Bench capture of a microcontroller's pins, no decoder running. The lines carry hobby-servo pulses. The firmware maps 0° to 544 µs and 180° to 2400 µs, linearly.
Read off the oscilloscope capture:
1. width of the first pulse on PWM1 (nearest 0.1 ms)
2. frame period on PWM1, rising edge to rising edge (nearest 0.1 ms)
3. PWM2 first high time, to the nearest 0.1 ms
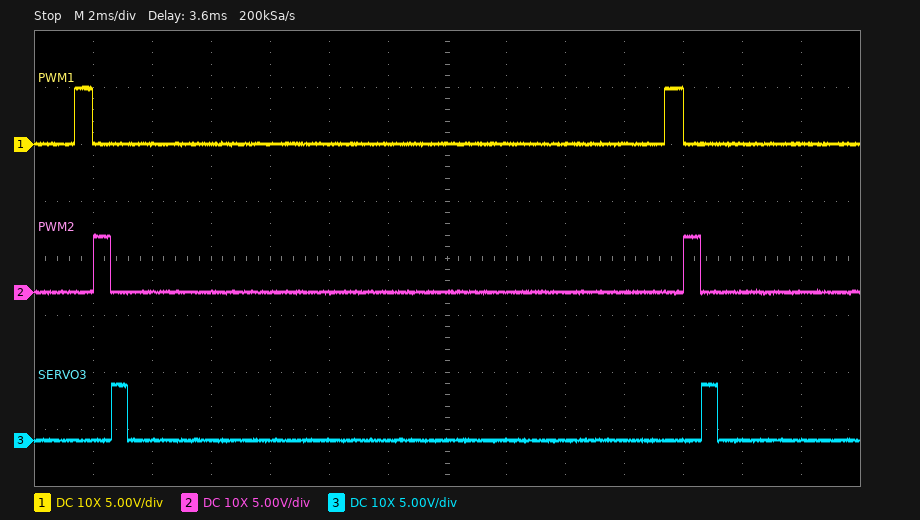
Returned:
0.6 ms
20.0 ms
0.6 ms
